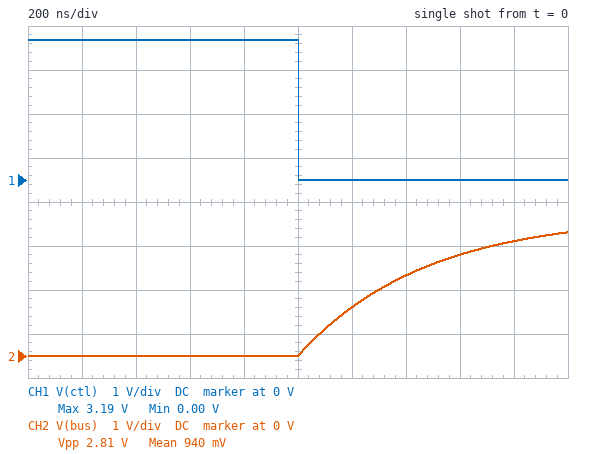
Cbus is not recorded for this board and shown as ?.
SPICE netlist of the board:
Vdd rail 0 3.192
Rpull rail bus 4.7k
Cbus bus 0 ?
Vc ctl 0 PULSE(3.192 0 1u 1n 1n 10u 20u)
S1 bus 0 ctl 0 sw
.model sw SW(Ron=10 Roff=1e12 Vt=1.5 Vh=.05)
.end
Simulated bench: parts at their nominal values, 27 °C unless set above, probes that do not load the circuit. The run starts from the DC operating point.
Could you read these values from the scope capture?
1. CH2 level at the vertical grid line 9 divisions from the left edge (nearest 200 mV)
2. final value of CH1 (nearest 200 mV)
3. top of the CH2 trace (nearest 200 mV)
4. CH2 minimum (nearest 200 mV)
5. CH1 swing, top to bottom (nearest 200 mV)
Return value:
2.6 V
0 V
2.8 V
0 V
3.2 V
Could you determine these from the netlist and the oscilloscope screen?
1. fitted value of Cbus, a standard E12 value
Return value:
100 pF
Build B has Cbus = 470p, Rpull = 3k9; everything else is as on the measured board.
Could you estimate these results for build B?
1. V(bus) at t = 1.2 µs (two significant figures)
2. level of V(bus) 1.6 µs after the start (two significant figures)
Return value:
340 mV
900 mV
